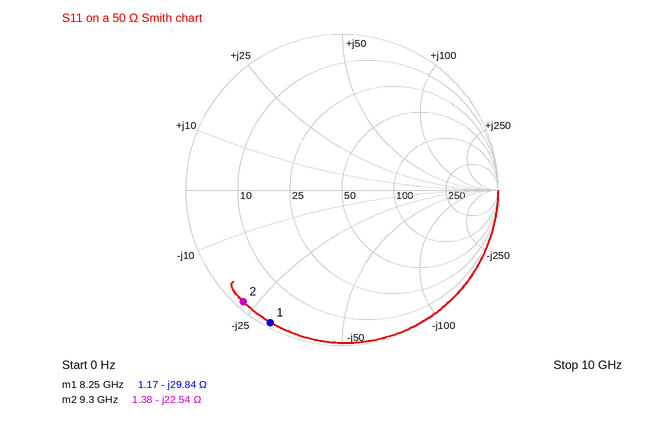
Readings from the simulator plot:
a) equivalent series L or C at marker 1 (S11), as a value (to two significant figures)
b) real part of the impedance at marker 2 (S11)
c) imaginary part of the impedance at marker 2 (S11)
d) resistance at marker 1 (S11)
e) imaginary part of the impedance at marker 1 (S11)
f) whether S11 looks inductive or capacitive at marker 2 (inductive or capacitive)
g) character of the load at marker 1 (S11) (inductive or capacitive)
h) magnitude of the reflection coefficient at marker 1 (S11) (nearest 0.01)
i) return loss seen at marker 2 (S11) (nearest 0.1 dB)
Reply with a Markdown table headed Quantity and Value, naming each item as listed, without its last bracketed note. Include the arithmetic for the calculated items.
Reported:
| Quantity | Value |
|---|---|
| equivalent series L or C at marker 1 (S11), as a value | C = 1/(2π × 8.25 GHz × 29.84 Ω) ≈ 646 fF, so 650 fF to two significant figures |
| real part of the impedance at marker 2 | 1.38 Ω |
| imaginary part of the impedance at marker 2 | -22.54 Ω |
| resistance at marker 1 | 1.17 Ω |
| imaginary part of the impedance at marker 1 | -29.84 Ω |
| whether S11 looks inductive or capacitive at marker 2 | capacitive |
| character of the load at marker 1 (S11) | capacitive |
| magnitude of the reflection coefficient at marker 1 (S11) | 0.97 |
| return loss seen at marker 2 (S11) | 0.4 dB |
